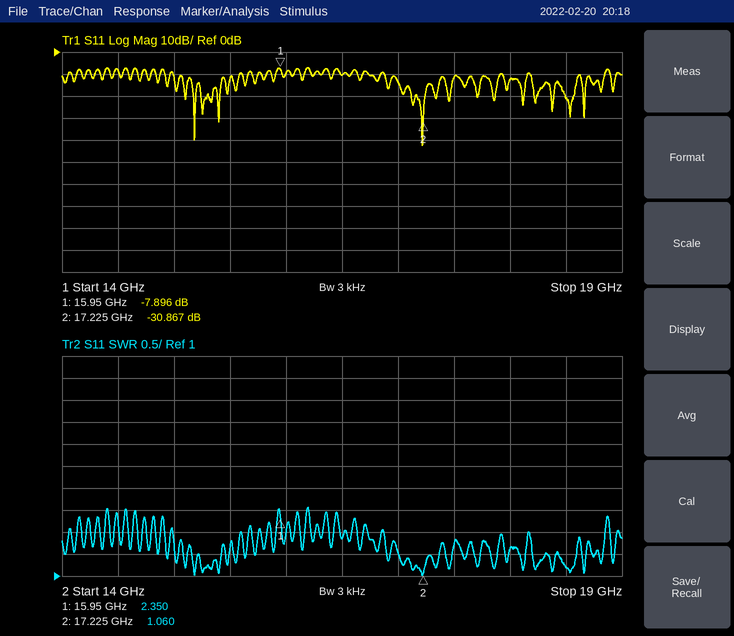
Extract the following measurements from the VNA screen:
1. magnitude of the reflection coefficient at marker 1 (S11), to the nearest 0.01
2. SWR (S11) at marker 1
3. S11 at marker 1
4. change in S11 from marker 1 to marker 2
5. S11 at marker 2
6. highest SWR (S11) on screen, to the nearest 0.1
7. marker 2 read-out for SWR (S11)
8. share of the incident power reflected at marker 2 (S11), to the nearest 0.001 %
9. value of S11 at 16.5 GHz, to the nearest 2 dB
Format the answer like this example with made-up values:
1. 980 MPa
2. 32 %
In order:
1. 0.40
2. 2.350
3. -7.896 dB
4. -22.971 dB
5. -30.867 dB
6. 2.6
7. 1.060
8. 0.082 %
9. -10 dB
